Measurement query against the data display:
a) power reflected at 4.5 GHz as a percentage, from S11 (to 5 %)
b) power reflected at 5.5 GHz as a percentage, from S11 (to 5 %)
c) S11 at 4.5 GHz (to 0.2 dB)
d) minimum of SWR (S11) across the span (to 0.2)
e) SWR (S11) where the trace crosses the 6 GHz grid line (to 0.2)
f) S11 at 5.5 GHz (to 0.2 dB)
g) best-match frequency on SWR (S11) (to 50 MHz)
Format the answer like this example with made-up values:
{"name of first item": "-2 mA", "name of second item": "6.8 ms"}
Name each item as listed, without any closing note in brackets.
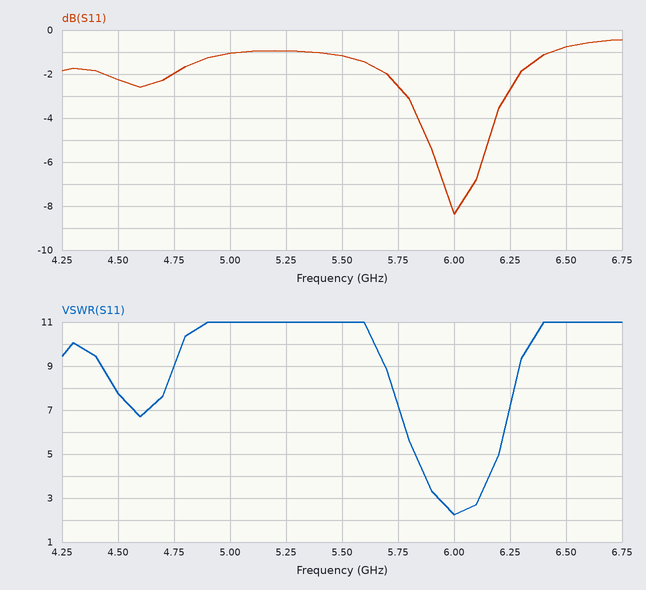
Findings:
{"power reflected at 4.5 GHz as a percentage, from S11": "60 %", "power reflected at 5.5 GHz as a percentage, from S11": "75 %", "S11 at 4.5 GHz": "-2.2 dB", "minimum of SWR (S11) across the span": "2.2", "SWR (S11) where the trace crosses the 6 GHz grid line": "2.2", "S11 at 5.5 GHz": "-1.2 dB", "best-match frequency on SWR (S11)": "6.00 GHz"}
